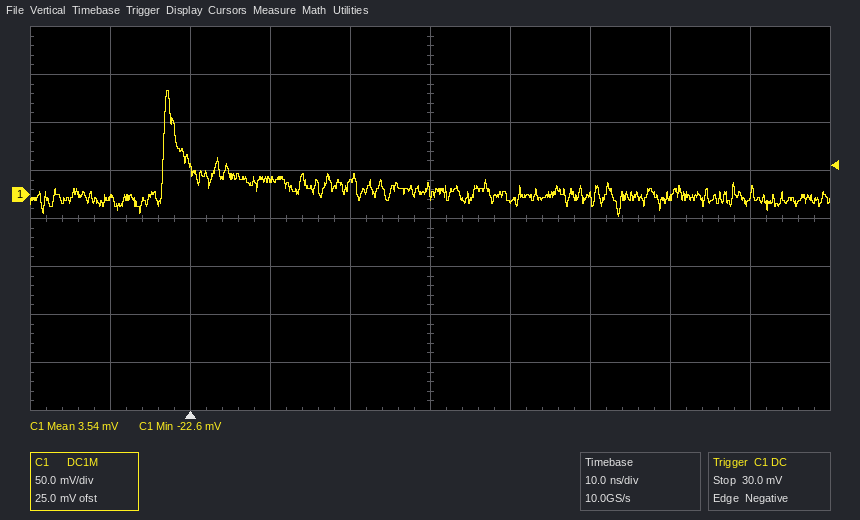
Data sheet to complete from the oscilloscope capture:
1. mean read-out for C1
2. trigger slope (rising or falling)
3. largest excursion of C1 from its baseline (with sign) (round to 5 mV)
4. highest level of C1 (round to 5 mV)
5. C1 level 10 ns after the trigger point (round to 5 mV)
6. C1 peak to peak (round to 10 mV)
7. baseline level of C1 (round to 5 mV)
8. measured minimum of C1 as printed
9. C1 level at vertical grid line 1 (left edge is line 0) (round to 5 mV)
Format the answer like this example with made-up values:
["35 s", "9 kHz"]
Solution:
["3.54 mV", "falling", "+110 mV", "110 mV", "15 mV", "130 mV", "0 mV", "-22.6 mV", "-5 mV"]
